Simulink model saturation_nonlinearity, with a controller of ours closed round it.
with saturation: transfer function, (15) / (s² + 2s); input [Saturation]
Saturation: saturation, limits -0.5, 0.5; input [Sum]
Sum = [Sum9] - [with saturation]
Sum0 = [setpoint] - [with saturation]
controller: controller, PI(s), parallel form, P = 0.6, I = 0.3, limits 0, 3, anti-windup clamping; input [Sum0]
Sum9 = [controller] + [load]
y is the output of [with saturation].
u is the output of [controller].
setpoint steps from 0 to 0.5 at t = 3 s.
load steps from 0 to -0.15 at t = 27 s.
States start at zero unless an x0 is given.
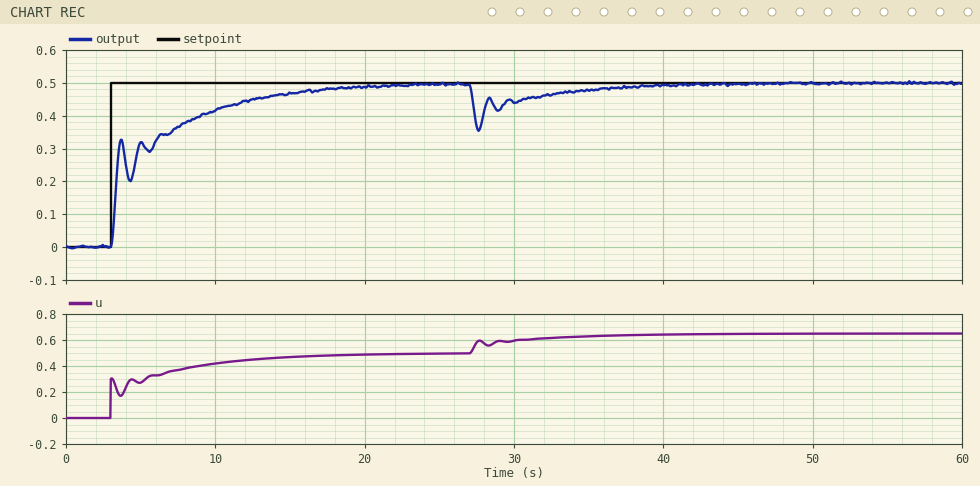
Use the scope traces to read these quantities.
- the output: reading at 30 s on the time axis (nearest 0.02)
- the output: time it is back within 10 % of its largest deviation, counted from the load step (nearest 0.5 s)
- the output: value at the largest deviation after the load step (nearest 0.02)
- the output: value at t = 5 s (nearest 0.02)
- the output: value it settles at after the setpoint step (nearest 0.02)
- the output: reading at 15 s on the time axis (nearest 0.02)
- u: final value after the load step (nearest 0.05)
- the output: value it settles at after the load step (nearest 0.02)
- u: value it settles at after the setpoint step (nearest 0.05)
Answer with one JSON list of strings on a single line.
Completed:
["0.44", "10.5 s", "0.36", "0.32", "0.50", "0.46", "0.65", "0.50", "0.50"]
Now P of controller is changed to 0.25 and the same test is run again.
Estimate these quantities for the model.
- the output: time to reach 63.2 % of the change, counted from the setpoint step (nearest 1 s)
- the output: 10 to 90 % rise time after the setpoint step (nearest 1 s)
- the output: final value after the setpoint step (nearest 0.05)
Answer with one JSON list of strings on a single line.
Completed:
["3 s", "8 s", "0.50"]
